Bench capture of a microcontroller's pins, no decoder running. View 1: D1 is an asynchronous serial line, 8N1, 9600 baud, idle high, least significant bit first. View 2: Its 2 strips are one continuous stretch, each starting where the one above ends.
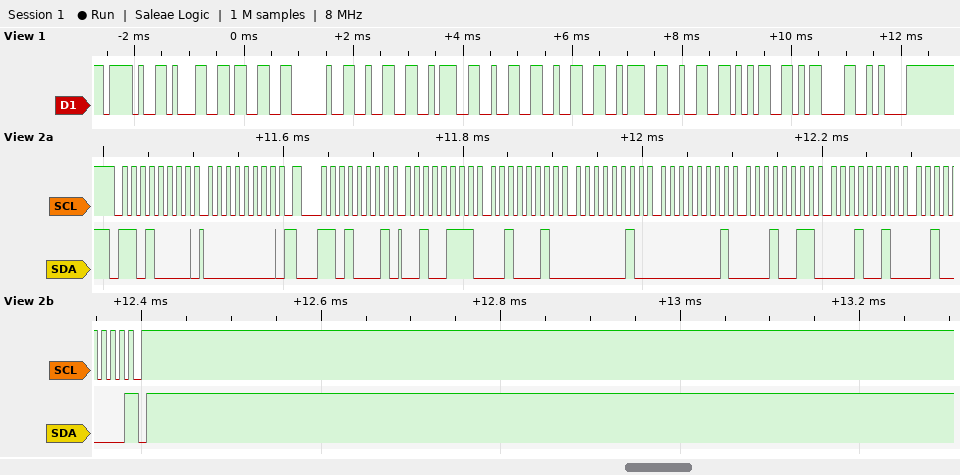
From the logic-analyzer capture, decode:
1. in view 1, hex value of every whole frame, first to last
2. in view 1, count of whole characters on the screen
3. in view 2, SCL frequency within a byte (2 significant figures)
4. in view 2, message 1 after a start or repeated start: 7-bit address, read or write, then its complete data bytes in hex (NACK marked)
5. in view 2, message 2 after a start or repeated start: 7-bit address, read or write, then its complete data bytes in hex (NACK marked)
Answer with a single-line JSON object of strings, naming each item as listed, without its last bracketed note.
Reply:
{"in view 1, hex value of every whole frame, first to last": "2F 31 33 20 32 3A 32 32 3A 32 35 0D 0A", "in view 1, count of whole characters on the screen": "13", "in view 2, SCL frequency within a byte": "100 kHz", "in view 2, message 1 after a start or repeated start: 7-bit address, read or write, then its complete data bytes in hex": "0x68 write: 00", "in view 2, message 2 after a start or repeated start: 7-bit address, read or write, then its complete data bytes in hex": "0x68 read: 27 22 02 01 13 12 20 NACK"}
